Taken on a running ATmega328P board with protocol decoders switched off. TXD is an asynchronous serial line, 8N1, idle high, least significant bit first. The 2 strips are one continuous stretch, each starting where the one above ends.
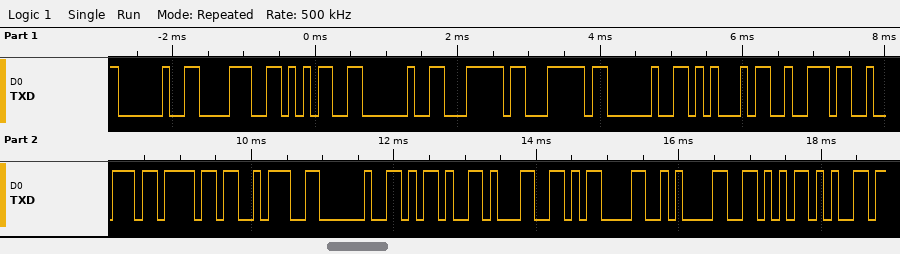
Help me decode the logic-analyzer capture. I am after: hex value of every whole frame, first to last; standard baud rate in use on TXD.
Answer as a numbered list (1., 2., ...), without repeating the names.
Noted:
1. 0x20 0x38 0x35 0x20 0x7C 0x7C 0x20 0x45 0x72 0x72 0x6F 0x3A 0x20 0x2D 0x31 0x0D 0x0A 0x56 0x65
2. 9600 baud
